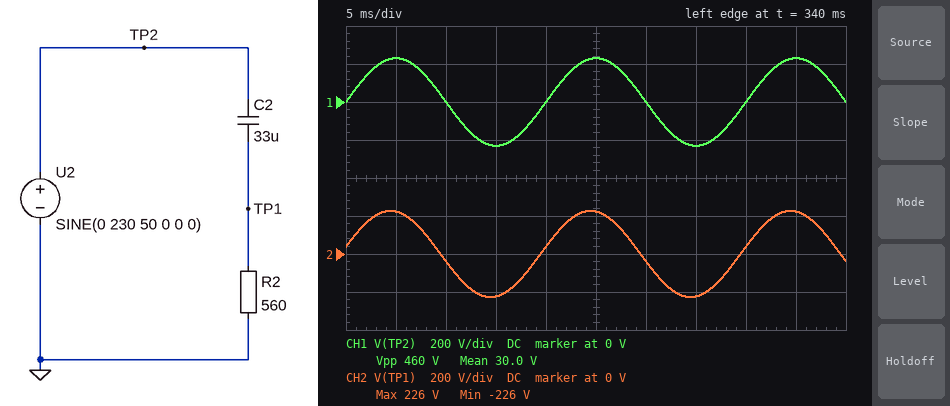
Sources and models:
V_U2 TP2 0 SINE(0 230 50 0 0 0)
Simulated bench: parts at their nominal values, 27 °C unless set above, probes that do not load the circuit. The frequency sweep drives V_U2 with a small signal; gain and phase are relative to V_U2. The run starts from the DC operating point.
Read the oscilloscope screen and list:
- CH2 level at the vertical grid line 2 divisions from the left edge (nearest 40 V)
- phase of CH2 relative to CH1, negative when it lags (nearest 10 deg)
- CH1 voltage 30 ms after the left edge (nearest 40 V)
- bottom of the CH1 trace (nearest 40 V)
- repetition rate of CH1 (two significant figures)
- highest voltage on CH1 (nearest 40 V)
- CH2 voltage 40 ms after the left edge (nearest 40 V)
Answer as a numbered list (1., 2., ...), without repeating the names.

1. -40 V
2. 10 deg
3. 0 V
4. -240 V
5. 50 Hz
6. 240 V
7. 40 V
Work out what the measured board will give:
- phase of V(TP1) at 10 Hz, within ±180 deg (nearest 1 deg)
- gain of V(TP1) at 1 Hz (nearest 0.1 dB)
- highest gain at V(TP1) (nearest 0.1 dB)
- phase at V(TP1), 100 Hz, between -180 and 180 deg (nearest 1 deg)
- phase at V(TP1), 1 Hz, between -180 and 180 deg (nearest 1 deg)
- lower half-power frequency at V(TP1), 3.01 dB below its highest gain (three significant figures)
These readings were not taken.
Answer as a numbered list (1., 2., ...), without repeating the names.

1. 41 deg
2. -18.8 dB
3. 0 dB
4. 5 deg
5. 83 deg
6. 8.61 Hz
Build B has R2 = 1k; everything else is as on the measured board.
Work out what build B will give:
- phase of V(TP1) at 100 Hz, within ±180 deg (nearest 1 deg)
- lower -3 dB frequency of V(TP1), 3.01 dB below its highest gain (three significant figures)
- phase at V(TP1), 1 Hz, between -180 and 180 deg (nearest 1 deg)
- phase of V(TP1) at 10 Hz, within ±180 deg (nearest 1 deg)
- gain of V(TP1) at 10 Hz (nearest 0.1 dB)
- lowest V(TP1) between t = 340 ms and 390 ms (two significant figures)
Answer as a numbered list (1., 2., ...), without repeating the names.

1. 3 deg
2. 4.82 Hz
3. 78 deg
4. 26 deg
5. -0.9 dB
6. -230 V
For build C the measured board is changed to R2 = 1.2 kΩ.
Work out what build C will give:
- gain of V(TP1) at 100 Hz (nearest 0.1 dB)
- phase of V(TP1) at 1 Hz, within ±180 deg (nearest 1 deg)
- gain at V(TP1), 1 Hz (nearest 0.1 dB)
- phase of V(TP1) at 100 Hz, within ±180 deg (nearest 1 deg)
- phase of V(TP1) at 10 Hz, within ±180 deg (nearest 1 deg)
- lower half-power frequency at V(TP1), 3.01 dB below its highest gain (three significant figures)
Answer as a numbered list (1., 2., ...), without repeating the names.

1. 0 dB
2. 76 deg
3. -12.3 dB
4. 2 deg
5. 22 deg
6. 4.02 Hz
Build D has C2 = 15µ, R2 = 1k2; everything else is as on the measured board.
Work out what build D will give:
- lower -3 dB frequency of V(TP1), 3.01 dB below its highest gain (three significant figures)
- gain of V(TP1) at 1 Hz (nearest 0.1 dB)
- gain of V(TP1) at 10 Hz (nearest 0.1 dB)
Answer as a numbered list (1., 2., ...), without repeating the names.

1. 8.84 Hz
2. -19.0 dB
3. -2.5 dB
